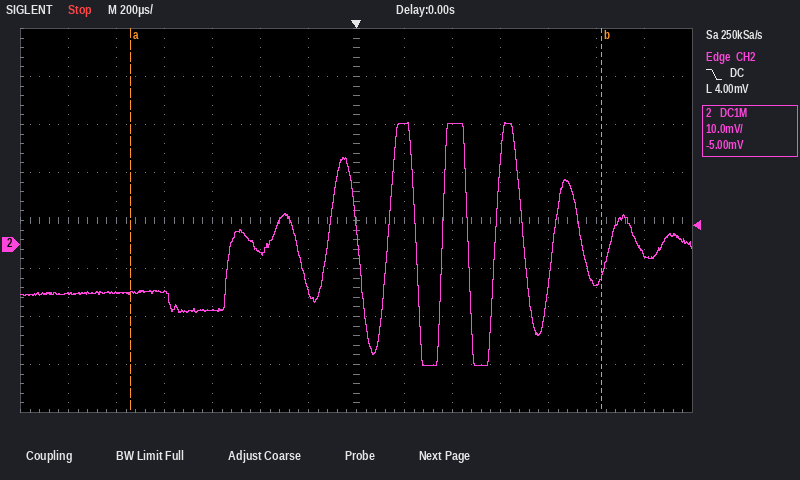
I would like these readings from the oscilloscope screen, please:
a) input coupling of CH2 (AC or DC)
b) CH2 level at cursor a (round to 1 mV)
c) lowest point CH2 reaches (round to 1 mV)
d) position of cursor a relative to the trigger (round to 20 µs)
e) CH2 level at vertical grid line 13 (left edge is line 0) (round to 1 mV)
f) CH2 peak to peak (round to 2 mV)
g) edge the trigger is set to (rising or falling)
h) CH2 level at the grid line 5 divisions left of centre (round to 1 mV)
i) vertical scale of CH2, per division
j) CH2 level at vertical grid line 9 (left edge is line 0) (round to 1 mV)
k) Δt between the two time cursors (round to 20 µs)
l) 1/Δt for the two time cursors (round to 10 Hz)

DC
-10 mV
-25 mV
-940 µs
-2 mV
50 mV
falling
-10 mV
10 mV
25 mV
1.96 ms
510 Hz
